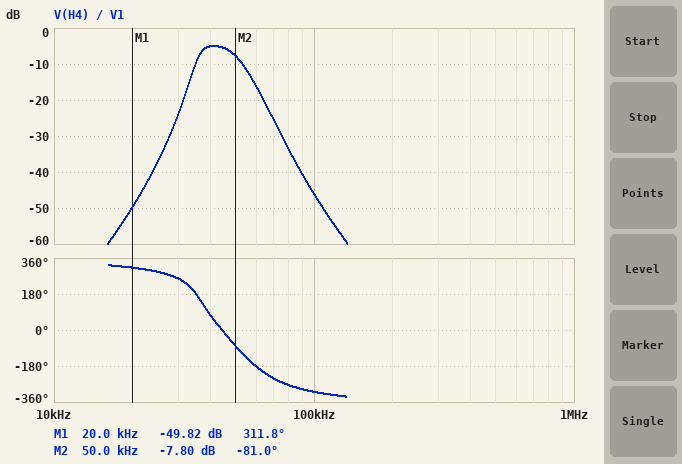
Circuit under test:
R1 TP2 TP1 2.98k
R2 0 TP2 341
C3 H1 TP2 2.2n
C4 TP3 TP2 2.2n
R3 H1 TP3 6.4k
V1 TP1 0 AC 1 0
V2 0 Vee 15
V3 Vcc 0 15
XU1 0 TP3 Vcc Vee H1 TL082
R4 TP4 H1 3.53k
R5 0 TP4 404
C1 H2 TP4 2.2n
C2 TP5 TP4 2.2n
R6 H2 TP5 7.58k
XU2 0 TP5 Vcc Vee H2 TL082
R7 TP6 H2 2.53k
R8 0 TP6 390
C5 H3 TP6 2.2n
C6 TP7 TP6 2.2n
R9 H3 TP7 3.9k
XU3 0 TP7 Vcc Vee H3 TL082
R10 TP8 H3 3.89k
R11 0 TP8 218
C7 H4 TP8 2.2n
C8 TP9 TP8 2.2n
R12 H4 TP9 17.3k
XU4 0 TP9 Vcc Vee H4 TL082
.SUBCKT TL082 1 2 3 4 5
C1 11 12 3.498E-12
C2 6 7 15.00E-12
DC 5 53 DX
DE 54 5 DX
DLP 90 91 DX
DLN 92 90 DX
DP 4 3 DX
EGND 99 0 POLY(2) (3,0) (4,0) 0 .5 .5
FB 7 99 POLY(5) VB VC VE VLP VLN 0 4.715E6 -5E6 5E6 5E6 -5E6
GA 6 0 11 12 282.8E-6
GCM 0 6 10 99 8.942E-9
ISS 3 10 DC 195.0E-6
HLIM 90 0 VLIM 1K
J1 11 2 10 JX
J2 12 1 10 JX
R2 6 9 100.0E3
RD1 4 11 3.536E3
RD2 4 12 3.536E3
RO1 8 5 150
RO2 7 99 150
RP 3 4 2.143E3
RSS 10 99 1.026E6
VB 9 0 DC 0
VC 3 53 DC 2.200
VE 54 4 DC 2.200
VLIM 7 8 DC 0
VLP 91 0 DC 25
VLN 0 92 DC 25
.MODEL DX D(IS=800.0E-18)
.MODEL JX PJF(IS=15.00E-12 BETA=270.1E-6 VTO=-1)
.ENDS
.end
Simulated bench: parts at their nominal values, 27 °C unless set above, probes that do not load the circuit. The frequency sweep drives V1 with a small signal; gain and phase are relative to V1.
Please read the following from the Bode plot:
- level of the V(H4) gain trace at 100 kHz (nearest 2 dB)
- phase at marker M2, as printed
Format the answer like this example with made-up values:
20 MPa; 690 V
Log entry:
-46 dB; -81.0 deg
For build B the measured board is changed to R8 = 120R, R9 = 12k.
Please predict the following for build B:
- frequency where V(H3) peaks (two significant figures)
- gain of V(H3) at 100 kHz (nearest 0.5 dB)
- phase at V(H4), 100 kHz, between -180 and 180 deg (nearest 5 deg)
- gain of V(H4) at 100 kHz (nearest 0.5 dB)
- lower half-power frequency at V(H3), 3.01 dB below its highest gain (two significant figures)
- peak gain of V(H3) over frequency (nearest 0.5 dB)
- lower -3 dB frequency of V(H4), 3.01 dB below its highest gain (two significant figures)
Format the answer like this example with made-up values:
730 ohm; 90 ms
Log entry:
55 kHz; -32.5 dB; 30 deg; -46.5 dB; 48 kHz; 4.5 dB; 38 kHz
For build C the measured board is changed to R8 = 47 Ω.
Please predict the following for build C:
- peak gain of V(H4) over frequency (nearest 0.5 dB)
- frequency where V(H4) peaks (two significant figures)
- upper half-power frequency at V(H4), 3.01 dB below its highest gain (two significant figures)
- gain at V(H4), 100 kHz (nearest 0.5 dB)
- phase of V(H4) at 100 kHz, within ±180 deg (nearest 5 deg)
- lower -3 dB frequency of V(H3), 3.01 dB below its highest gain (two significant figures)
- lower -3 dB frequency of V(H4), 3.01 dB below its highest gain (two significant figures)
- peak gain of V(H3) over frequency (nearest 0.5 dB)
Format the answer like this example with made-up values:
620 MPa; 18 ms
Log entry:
-25.0 dB; 40 kHz; 49 kHz; -51.5 dB; -170 deg; 41 kHz; 36 kHz; -25.5 dB
